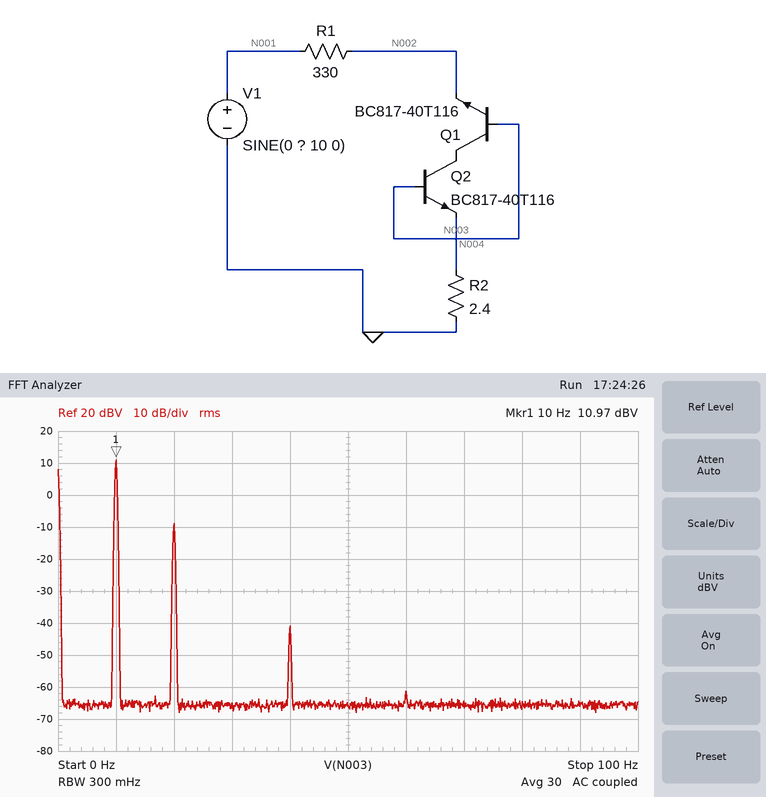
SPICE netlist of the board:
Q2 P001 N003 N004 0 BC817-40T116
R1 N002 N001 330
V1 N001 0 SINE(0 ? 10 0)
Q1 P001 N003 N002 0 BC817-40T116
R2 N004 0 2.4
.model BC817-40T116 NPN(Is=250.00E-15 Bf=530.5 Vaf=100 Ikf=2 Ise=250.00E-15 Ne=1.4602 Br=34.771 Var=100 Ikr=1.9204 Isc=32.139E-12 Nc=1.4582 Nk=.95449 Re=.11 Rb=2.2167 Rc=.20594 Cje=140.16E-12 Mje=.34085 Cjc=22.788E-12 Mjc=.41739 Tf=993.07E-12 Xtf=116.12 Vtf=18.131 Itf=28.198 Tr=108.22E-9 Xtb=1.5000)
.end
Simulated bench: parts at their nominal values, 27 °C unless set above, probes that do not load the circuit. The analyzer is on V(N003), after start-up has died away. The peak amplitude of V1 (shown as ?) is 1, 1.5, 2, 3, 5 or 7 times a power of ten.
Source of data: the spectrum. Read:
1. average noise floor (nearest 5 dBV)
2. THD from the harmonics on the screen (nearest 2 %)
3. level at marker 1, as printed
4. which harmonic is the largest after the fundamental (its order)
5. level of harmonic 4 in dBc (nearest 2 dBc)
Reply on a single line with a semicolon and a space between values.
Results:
-65 dBV; 10 %; 10.97 dBV; 2; -52 dBc
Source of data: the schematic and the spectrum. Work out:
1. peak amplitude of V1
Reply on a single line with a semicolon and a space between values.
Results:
10 V
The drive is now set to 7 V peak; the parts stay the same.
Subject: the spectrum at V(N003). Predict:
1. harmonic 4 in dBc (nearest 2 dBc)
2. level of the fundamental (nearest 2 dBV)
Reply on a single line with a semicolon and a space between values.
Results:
-54 dBc; 8 dBV
